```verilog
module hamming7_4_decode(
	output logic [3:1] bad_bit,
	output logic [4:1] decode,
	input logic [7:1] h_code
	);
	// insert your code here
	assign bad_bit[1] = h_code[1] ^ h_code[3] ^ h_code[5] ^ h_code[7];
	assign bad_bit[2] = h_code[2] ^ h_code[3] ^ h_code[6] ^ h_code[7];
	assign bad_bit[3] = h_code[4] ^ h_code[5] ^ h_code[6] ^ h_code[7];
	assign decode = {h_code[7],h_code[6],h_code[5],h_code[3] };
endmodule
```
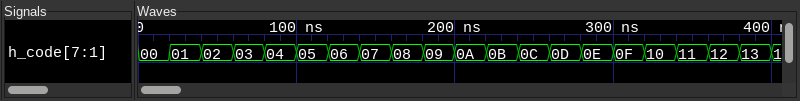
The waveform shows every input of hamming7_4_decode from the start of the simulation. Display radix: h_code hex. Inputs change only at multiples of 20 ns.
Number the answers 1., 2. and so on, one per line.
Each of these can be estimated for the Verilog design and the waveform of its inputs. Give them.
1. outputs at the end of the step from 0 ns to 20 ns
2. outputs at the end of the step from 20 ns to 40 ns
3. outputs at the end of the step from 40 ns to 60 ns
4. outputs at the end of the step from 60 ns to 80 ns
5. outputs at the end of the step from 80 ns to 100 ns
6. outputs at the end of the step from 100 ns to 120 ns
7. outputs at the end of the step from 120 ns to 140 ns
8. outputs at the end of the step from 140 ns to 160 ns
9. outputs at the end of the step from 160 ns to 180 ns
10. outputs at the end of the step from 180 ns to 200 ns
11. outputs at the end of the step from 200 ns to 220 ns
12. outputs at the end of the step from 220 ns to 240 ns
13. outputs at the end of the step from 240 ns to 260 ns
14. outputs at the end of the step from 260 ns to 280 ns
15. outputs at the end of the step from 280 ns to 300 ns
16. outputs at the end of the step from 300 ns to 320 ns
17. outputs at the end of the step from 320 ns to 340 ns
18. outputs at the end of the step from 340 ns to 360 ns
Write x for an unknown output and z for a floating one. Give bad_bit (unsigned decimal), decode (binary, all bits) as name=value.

1. bad_bit=0, decode=0000
2. bad_bit=1, decode=0000
3. bad_bit=2, decode=0000
4. bad_bit=3, decode=0000
5. bad_bit=3, decode=0001
6. bad_bit=2, decode=0001
7. bad_bit=1, decode=0001
8. bad_bit=0, decode=0001
9. bad_bit=4, decode=0000
10. bad_bit=5, decode=0000
11. bad_bit=6, decode=0000
12. bad_bit=7, decode=0000
13. bad_bit=7, decode=0001
14. bad_bit=6, decode=0001
15. bad_bit=5, decode=0001
16. bad_bit=4, decode=0001
17. bad_bit=5, decode=0010
18. bad_bit=4, decode=0010
